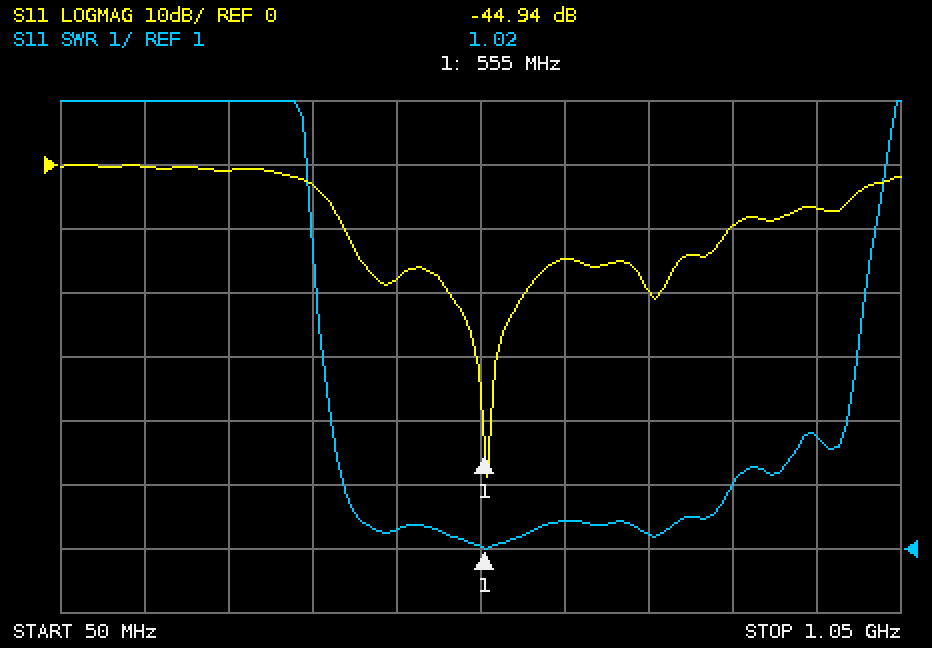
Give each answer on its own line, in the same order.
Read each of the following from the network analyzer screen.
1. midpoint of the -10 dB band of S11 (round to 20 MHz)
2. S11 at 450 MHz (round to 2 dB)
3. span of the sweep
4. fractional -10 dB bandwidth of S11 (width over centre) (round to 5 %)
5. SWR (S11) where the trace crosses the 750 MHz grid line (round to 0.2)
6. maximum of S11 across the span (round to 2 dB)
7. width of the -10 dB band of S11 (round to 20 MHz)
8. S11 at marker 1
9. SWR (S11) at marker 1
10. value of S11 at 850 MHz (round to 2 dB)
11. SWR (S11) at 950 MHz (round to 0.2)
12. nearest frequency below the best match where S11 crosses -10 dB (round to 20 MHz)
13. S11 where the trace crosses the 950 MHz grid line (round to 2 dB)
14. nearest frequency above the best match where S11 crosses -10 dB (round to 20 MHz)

620 MHz
-18 dB
1 GHz
75 %
1.2
0 dB
460 MHz
-44.94 dB
1.02
-10 dB
2.8
380 MHz
-6 dB
840 MHz
